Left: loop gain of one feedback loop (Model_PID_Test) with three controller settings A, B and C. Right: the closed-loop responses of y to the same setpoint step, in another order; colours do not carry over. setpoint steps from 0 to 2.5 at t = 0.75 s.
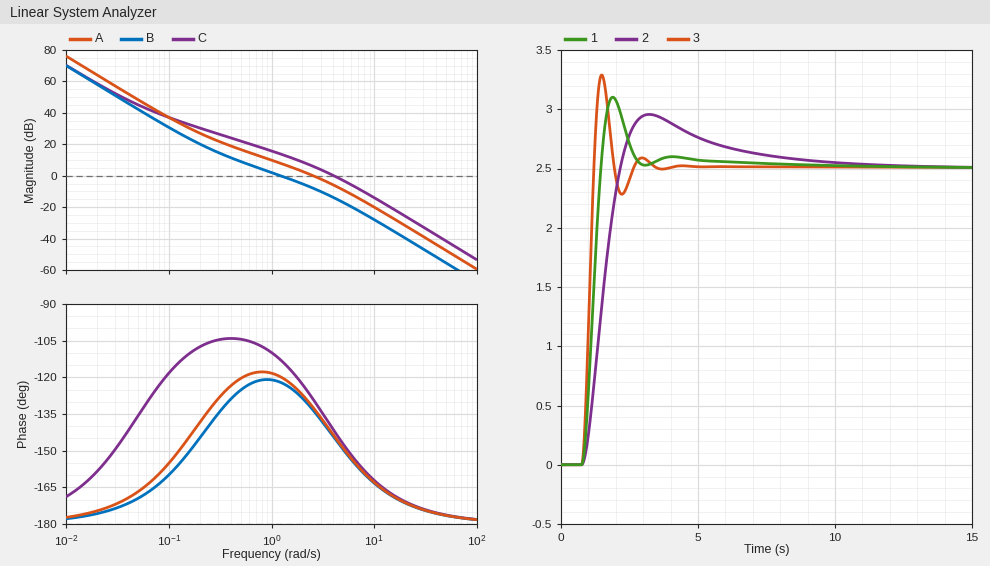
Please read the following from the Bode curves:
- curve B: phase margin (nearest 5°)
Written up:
60°
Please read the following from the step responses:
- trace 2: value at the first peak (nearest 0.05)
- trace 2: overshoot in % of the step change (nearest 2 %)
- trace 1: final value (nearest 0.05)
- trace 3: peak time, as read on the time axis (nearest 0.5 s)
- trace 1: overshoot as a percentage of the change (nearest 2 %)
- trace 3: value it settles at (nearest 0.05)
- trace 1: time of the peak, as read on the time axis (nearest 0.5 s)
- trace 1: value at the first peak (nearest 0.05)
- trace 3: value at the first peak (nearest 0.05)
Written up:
2.95
18 %
2.50
1.5 s
24 %
2.50
2.0 s
3.10
3.30
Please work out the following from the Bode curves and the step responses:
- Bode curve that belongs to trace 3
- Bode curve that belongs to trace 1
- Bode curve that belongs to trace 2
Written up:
C
A
B
